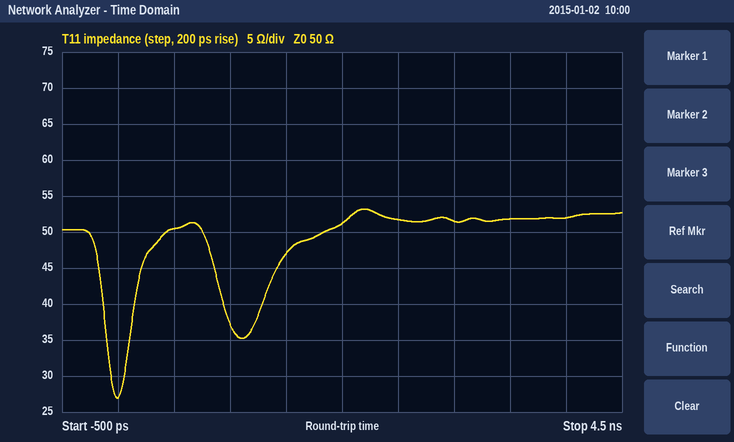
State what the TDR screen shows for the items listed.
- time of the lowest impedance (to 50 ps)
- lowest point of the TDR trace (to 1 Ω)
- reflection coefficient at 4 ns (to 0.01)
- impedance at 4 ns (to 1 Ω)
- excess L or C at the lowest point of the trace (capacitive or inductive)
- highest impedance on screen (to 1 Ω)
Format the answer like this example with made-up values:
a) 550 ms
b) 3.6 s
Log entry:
a) 0 ps
b) 27 Ω
c) +0.02
d) 52 Ω
e) capacitive
f) 53 Ω
